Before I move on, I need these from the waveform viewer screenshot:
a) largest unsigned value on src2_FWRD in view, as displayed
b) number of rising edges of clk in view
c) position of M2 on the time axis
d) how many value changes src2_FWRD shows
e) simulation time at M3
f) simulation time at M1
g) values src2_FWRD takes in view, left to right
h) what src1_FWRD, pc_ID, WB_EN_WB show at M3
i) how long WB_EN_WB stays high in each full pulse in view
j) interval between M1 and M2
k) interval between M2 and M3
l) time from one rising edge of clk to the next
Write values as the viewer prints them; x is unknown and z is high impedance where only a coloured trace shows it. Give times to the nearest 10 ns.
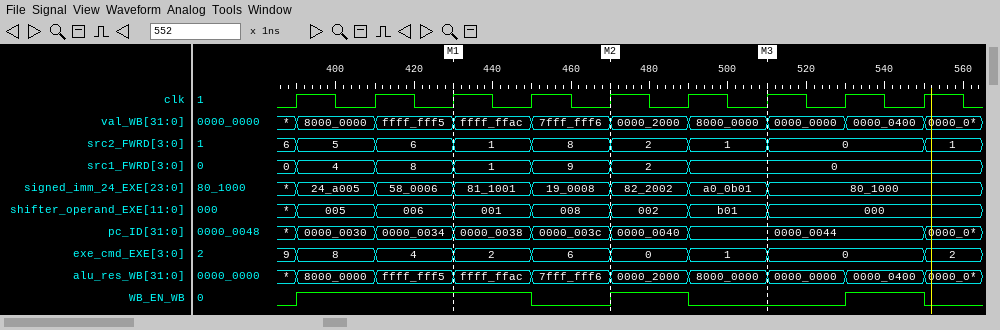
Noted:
8
9
470 ns
8
510 ns
430 ns
6, 5, 6, 1, 8, 2, 1, 0, 1
src1_FWRD=0, pc_ID=0000_0044, WB_EN_WB=0
60 ns, 20 ns, 20 ns
40 ns
40 ns
20 ns
